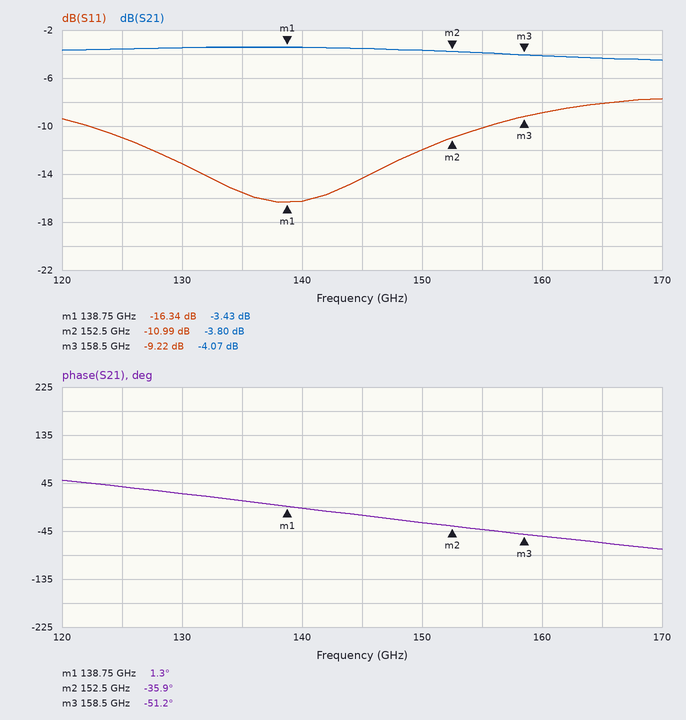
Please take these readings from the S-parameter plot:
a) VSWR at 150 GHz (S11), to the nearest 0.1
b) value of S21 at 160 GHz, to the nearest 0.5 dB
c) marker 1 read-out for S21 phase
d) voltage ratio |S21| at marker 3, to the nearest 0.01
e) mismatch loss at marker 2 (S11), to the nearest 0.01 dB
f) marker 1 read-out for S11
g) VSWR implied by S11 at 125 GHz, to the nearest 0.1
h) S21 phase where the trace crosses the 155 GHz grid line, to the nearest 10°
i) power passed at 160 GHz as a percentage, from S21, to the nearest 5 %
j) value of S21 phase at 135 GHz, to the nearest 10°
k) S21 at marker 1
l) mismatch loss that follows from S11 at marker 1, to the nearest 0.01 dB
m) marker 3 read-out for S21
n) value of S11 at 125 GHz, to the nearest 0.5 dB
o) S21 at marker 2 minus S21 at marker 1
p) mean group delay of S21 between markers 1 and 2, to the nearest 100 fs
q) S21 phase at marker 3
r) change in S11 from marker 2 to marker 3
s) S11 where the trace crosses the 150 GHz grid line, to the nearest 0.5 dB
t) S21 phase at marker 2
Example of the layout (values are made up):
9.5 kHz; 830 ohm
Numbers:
1.7; -4.0 dB; 1.3°; 0.63; 0.36 dB; -16.34 dB; 1.8; -40°; 40 %; 10°; -3.43 dB; 0.10 dB; -4.07 dB; -11.0 dB; -0.37 dB; 7.5 ps; -51.2°; 1.77 dB; -12.0 dB; -35.9°
